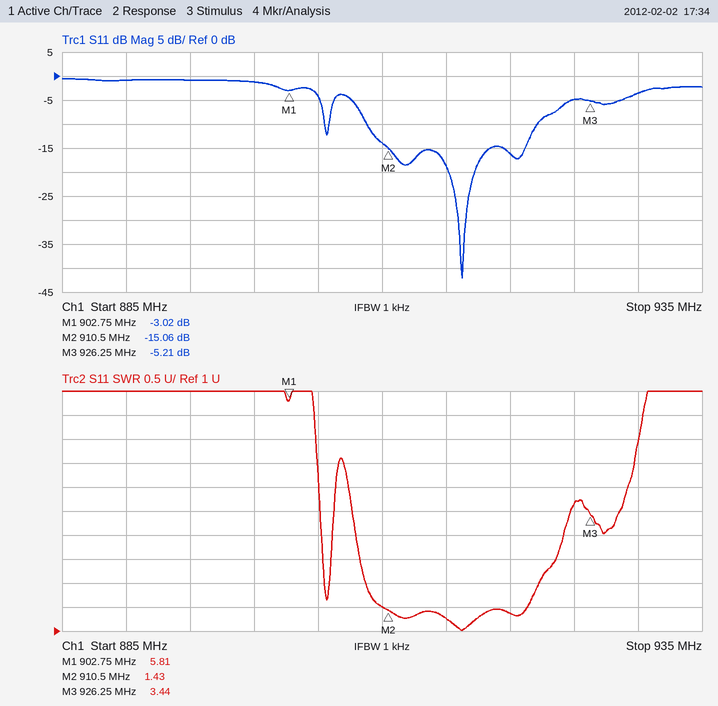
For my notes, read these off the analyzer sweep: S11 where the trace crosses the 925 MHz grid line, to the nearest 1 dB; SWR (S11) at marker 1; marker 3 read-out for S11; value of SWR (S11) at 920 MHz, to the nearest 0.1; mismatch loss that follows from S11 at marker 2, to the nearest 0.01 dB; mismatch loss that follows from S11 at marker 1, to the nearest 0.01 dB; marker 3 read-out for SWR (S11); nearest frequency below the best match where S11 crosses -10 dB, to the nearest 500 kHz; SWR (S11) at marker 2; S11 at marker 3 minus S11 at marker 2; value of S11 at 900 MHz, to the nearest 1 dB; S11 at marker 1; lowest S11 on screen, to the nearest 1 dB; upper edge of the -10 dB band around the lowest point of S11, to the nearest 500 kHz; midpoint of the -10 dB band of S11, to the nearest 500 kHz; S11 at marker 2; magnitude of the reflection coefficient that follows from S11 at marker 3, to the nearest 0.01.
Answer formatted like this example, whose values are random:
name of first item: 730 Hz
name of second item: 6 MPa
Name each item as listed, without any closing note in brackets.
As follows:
S11 where the trace crosses the 925 MHz grid line, to the nearest 1 dB: -5 dB
SWR (S11) at marker 1: 5.81
marker 3 read-out for S11: -5.21 dB
value of SWR (S11) at 920 MHz, to the nearest 0.1: 1.4
mismatch loss that follows from S11 at marker 2, to the nearest 0.01 dB: 0.14 dB
mismatch loss that follows from S11 at marker 1, to the nearest 0.01 dB: 3.00 dB
marker 3 read-out for SWR: 3.44
nearest frequency below the best match where S11 crosses -10 dB, to the nearest 500 kHz: 909.0 MHz
SWR (S11) at marker 2: 1.43
S11 at marker 3 minus S11 at marker 2: 9.85 dB
value of S11 at 900 MHz, to the nearest 1 dB: -1 dB
S11 at marker 1: -3.02 dB
lowest S11 on screen, to the nearest 1 dB: -42 dB
upper edge of the -10 dB band around the lowest point of S11, to the nearest 500 kHz: 922.0 MHz
midpoint of the -10 dB band of S11, to the nearest 500 kHz: 915.5 MHz
S11 at marker 2: -15.06 dB
magnitude of the reflection coefficient that follows from S11 at marker 3, to the nearest 0.01: 0.55
